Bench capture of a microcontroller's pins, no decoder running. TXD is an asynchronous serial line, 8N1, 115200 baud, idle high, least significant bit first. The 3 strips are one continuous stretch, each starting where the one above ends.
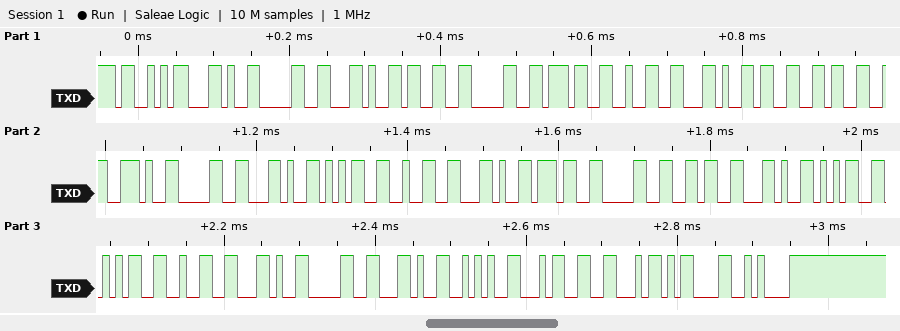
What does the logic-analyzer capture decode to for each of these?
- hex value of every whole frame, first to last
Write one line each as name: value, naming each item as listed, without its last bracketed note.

hex value of every whole frame, first to last: 53 2C 30 2C 33 30 37 32 2C 33 33 2E 30 2C 35 32 2C 37 30 36 2C 35 35 32 2C 30 2C 2A 34 46 0D 0A
